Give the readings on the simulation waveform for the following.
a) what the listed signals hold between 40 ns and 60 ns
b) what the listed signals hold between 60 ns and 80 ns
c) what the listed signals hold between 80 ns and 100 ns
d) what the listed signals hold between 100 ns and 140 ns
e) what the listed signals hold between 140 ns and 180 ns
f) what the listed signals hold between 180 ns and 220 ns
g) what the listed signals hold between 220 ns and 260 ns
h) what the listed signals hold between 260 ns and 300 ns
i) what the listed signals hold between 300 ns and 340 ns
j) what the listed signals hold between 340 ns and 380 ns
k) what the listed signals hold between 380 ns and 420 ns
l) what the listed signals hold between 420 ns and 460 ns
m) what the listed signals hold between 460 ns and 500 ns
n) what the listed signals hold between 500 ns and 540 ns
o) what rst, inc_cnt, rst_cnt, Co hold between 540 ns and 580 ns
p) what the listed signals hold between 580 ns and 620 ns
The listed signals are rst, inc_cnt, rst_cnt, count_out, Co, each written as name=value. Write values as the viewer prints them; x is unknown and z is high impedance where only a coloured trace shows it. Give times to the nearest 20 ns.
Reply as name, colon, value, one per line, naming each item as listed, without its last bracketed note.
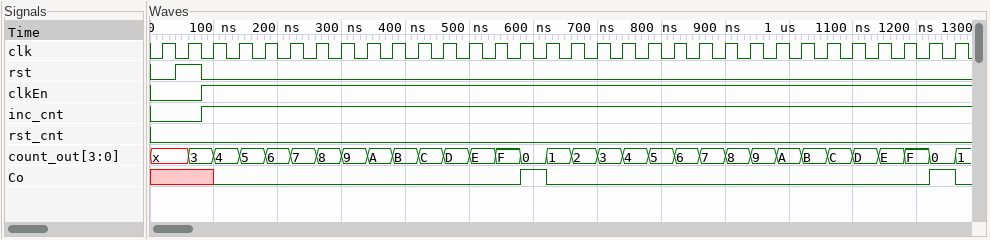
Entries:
what the listed signals hold between 40 ns and 60 ns: rst=1, inc_cnt=0, rst_cnt=0, count_out=x, Co=x
what the listed signals hold between 60 ns and 80 ns: rst=1, inc_cnt=0, rst_cnt=0, count_out=3, Co=x
what the listed signals hold between 80 ns and 100 ns: rst=0, inc_cnt=1, rst_cnt=0, count_out=3, Co=x
what the listed signals hold between 100 ns and 140 ns: rst=0, inc_cnt=1, rst_cnt=0, count_out=4, Co=0
what the listed signals hold between 140 ns and 180 ns: rst=0, inc_cnt=1, rst_cnt=0, count_out=5, Co=0
what the listed signals hold between 180 ns and 220 ns: rst=0, inc_cnt=1, rst_cnt=0, count_out=6, Co=0
what the listed signals hold between 220 ns and 260 ns: rst=0, inc_cnt=1, rst_cnt=0, count_out=7, Co=0
what the listed signals hold between 260 ns and 300 ns: rst=0, inc_cnt=1, rst_cnt=0, count_out=8, Co=0
what the listed signals hold between 300 ns and 340 ns: rst=0, inc_cnt=1, rst_cnt=0, count_out=9, Co=0
what the listed signals hold between 340 ns and 380 ns: rst=0, inc_cnt=1, rst_cnt=0, count_out=A, Co=0
what the listed signals hold between 380 ns and 420 ns: rst=0, inc_cnt=1, rst_cnt=0, count_out=B, Co=0
what the listed signals hold between 420 ns and 460 ns: rst=0, inc_cnt=1, rst_cnt=0, count_out=C, Co=0
what the listed signals hold between 460 ns and 500 ns: rst=0, inc_cnt=1, rst_cnt=0, count_out=D, Co=0
what the listed signals hold between 500 ns and 540 ns: rst=0, inc_cnt=1, rst_cnt=0, count_out=E, Co=0
what rst, inc_cnt, rst_cnt, Co hold between 540 ns and 580 ns: rst=0, inc_cnt=1, rst_cnt=0, Co=0
what the listed signals hold between 580 ns and 620 ns: rst=0, inc_cnt=1, rst_cnt=0, count_out=0, Co=1
